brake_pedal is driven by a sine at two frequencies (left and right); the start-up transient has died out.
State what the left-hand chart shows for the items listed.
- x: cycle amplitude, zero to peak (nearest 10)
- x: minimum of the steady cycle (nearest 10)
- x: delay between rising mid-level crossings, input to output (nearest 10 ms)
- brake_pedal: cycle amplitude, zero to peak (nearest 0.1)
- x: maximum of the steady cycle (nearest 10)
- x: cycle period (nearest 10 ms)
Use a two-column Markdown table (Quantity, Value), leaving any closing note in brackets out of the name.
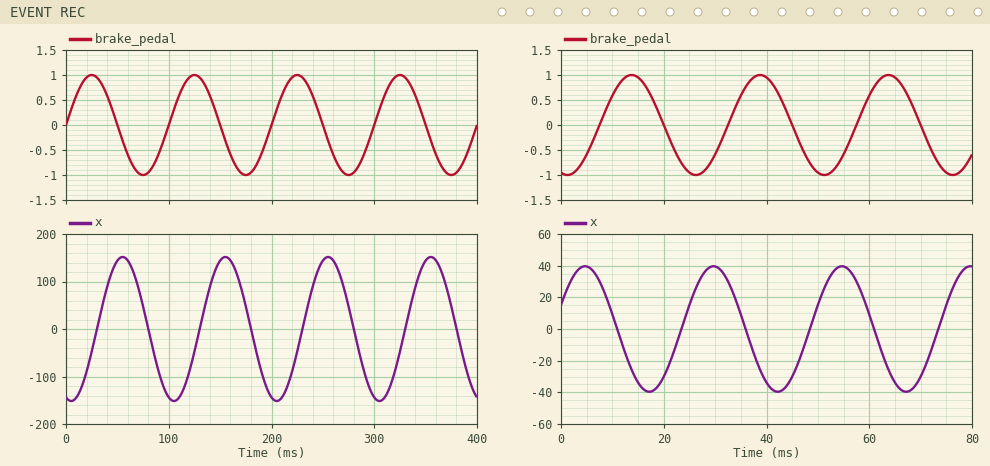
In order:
| Quantity | Value |
|---|---|
| x: cycle amplitude, zero to peak | 150 |
| x: minimum of the steady cycle | -150 |
| x: delay between rising mid-level crossings, input to output | 30 ms |
| brake_pedal: cycle amplitude, zero to peak | 1.0 |
| x: maximum of the steady cycle | 150 |
| x: cycle period | 100 ms |
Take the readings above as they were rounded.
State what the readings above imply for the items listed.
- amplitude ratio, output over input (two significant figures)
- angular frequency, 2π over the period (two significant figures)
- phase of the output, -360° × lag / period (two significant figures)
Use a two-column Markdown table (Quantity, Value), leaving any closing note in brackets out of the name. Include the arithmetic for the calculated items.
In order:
| Quantity | Value |
|---|---|
| amplitude ratio, output over input | 150 / 1 = 150 |
| angular frequency, 2π over the period | 2π / 100 = 0.063 rad/ms |
| phase of the output, -360° × lag / period | -360 × 30 / 100 = -110° |
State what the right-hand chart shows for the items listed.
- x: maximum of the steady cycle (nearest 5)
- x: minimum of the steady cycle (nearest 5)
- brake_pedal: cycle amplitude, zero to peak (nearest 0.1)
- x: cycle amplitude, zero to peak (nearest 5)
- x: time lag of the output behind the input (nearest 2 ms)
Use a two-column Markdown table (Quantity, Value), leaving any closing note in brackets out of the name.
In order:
| Quantity | Value |
|---|---|
| x: maximum of the steady cycle | 40 |
| x: minimum of the steady cycle | -40 |
| brake_pedal: cycle amplitude, zero to peak | 1.0 |
| x: cycle amplitude, zero to peak | 40 |
| x: time lag of the output behind the input | 16 ms |
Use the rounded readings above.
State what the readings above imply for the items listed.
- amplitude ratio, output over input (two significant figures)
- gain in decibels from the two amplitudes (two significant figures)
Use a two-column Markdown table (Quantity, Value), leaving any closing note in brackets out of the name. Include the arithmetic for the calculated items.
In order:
| Quantity | Value |
|---|---|
| amplitude ratio, output over input | 40 / 1 = 40 |
| gain in decibels from the two amplitudes | 20 log10(40 / 1) = 32 dB |
